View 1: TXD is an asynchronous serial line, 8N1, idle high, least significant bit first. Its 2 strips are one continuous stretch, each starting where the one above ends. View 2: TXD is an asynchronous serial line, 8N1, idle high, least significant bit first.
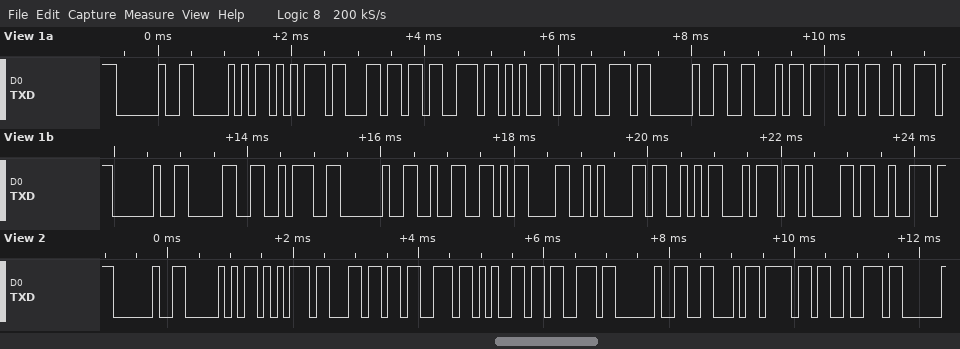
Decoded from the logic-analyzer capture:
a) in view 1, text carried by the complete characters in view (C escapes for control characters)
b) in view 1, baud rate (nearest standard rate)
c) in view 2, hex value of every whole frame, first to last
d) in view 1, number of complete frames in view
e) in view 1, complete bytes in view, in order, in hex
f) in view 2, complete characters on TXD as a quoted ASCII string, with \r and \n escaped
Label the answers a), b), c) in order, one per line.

a) " Pulses For 0: 2\r\nStar"
b) 9600 baud
c) 20 50 75 6C 73 65 73 20 46 6F 72
d) 22
e) 20 50 75 6C 73 65 73 20 46 6F 72 20 30 3A 20 32 0D 0A 53 74 61 72
f) " Pulses For"
